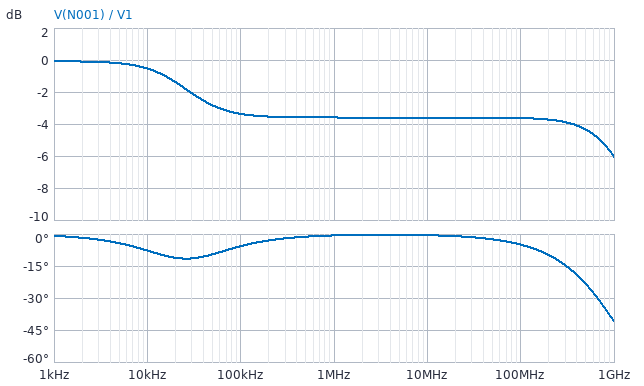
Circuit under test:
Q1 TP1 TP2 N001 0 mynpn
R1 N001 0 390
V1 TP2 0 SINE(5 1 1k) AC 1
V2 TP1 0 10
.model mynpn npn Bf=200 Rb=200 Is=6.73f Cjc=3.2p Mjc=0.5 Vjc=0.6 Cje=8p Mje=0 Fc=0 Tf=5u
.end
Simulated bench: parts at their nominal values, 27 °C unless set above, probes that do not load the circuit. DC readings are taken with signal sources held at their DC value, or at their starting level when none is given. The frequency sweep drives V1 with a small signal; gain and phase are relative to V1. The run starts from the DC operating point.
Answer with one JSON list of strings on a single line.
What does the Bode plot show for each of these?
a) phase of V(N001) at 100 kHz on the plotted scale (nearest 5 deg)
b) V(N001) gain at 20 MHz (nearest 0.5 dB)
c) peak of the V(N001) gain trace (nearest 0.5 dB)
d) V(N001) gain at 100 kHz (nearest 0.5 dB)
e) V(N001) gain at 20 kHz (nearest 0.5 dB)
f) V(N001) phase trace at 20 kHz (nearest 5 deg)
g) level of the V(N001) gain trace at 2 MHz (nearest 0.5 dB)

["-5 deg", "-3.5 dB", "0 dB", "-3.5 dB", "-1.5 dB", "-10 deg", "-3.5 dB"]
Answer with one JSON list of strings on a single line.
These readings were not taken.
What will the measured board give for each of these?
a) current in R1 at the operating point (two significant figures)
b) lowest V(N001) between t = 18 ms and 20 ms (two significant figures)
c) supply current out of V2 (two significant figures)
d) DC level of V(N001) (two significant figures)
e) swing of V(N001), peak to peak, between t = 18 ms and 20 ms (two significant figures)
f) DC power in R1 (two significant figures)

["11 mA", "3.3 V", "11 mA", "4.3 V", "2.0 V", "47 mW"]
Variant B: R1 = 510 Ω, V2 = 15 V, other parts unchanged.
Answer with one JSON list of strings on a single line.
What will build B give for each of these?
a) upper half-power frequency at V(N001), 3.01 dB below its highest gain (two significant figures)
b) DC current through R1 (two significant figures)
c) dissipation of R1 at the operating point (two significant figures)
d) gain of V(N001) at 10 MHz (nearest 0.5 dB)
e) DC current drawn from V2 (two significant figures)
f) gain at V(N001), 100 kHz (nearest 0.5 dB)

["320 MHz", "8.4 mA", "36 mW", "-3.0 dB", "8.3 mA", "-2.5 dB"]
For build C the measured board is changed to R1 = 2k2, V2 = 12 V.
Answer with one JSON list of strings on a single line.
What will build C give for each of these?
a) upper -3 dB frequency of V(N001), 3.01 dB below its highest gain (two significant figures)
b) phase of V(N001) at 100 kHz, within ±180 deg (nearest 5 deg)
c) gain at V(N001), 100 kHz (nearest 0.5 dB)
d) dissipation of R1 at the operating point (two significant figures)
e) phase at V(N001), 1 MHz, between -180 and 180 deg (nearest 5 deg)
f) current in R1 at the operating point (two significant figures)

["810 MHz", "0 deg", "-0.5 dB", "8.5 mW", "0 deg", "2.0 mA"]
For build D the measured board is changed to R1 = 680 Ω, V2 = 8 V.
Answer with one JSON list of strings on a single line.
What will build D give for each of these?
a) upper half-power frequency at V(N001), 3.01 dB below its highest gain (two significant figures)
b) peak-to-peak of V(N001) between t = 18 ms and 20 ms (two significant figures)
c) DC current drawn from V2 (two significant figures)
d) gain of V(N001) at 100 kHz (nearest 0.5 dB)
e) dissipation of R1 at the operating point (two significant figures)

["360 MHz", "2.0 V", "6.3 mA", "-2.0 dB", "27 mW"]
